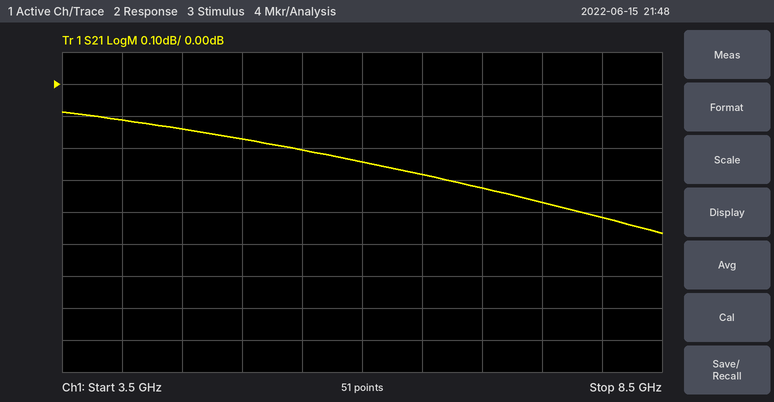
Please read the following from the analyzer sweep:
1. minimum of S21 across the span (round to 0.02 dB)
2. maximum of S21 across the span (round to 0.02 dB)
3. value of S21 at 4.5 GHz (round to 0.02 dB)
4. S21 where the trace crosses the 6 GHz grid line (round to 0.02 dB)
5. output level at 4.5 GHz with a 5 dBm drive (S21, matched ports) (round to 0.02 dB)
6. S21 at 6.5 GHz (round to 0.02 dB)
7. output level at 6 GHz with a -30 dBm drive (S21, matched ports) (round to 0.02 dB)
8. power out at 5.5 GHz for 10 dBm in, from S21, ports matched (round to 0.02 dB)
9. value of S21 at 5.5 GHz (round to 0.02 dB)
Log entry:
-0.46 dB
-0.08 dB
-0.14 dB
-0.24 dB
4.86 dBm
-0.28 dB
-30.24 dBm
9.80 dBm
-0.20 dB
